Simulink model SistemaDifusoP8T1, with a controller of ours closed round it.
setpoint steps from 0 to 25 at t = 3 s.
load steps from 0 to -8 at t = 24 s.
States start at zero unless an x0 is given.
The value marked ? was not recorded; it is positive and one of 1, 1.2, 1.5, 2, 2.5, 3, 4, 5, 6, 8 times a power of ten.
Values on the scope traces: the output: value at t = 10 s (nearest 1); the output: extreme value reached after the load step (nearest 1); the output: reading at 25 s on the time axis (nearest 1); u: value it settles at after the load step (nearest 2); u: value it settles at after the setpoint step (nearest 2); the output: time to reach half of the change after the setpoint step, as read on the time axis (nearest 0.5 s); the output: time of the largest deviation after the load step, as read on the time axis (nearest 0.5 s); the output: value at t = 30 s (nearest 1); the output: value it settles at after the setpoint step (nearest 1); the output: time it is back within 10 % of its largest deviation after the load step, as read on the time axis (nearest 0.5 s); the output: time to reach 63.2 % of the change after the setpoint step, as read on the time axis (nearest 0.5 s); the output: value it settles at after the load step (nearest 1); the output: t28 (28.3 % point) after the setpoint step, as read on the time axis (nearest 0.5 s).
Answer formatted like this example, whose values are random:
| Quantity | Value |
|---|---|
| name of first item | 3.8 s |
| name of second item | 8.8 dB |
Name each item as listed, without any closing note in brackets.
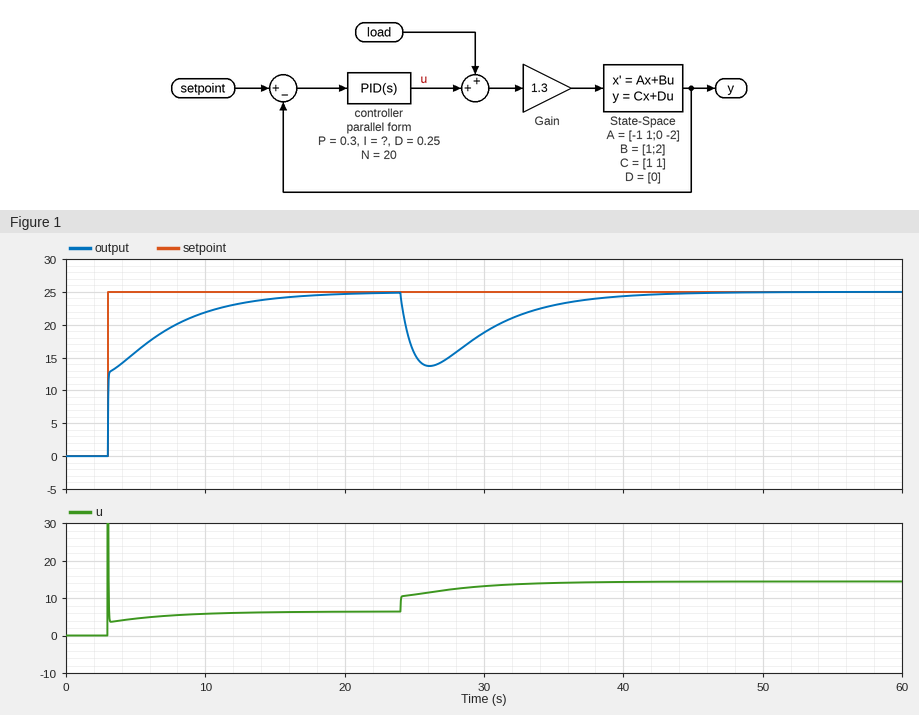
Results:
| Quantity | Value |
|---|---|
| the output: value at t = 10 s | 22 |
| the output: extreme value reached after the load step | 14 |
| the output: reading at 25 s on the time axis | 16 |
| u: value it settles at after the load step | 14 |
| u: value it settles at after the setpoint step | 6 |
| the output: time to reach half of the change after the setpoint step, as read on the time axis | 3.0 s |
| the output: time of the largest deviation after the load step, as read on the time axis | 26.0 s |
| the output: value at t = 30 s | 19 |
| the output: value it settles at after the setpoint step | 25 |
| the output: time it is back within 10 % of its largest deviation after the load step, as read on the time axis | 37.5 s |
| the output: time to reach 63.2 % of the change after the setpoint step, as read on the time axis | 5.0 s |
| the output: value it settles at after the load step | 25 |
| the output: t28 (28.3 % point) after the setpoint step, as read on the time axis | 3.0 s |
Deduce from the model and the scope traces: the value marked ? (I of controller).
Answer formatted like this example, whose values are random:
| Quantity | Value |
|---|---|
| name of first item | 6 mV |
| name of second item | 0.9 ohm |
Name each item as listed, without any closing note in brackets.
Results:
| Quantity | Value |
|---|---|
| the value marked ? | 0.1 |
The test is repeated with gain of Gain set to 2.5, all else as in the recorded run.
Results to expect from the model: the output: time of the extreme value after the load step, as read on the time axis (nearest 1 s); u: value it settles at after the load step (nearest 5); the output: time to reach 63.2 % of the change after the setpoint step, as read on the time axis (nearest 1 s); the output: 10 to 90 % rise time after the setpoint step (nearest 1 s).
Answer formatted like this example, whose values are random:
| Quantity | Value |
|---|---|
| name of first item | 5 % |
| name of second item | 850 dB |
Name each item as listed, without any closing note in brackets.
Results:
| Quantity | Value |
|---|---|
| the output: time of the extreme value after the load step, as read on the time axis | 26 s |
| u: value it settles at after the load step | 10 |
| the output: time to reach 63.2 % of the change after the setpoint step, as read on the time axis | 3 s |
| the output: 10 to 90 % rise time after the setpoint step | 5 s |
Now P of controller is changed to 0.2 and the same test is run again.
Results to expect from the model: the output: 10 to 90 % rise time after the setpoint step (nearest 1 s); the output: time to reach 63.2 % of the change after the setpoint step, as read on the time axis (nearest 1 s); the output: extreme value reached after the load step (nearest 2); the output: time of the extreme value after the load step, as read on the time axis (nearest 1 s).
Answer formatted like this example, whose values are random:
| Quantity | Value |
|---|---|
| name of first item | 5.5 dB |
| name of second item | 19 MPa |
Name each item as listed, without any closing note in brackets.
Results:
| Quantity | Value |
|---|---|
| the output: 10 to 90 % rise time after the setpoint step | 7 s |
| the output: time to reach 63.2 % of the change after the setpoint step, as read on the time axis | 6 s |
| the output: extreme value reached after the load step | 12 |
| the output: time of the extreme value after the load step, as read on the time axis | 26 s |
